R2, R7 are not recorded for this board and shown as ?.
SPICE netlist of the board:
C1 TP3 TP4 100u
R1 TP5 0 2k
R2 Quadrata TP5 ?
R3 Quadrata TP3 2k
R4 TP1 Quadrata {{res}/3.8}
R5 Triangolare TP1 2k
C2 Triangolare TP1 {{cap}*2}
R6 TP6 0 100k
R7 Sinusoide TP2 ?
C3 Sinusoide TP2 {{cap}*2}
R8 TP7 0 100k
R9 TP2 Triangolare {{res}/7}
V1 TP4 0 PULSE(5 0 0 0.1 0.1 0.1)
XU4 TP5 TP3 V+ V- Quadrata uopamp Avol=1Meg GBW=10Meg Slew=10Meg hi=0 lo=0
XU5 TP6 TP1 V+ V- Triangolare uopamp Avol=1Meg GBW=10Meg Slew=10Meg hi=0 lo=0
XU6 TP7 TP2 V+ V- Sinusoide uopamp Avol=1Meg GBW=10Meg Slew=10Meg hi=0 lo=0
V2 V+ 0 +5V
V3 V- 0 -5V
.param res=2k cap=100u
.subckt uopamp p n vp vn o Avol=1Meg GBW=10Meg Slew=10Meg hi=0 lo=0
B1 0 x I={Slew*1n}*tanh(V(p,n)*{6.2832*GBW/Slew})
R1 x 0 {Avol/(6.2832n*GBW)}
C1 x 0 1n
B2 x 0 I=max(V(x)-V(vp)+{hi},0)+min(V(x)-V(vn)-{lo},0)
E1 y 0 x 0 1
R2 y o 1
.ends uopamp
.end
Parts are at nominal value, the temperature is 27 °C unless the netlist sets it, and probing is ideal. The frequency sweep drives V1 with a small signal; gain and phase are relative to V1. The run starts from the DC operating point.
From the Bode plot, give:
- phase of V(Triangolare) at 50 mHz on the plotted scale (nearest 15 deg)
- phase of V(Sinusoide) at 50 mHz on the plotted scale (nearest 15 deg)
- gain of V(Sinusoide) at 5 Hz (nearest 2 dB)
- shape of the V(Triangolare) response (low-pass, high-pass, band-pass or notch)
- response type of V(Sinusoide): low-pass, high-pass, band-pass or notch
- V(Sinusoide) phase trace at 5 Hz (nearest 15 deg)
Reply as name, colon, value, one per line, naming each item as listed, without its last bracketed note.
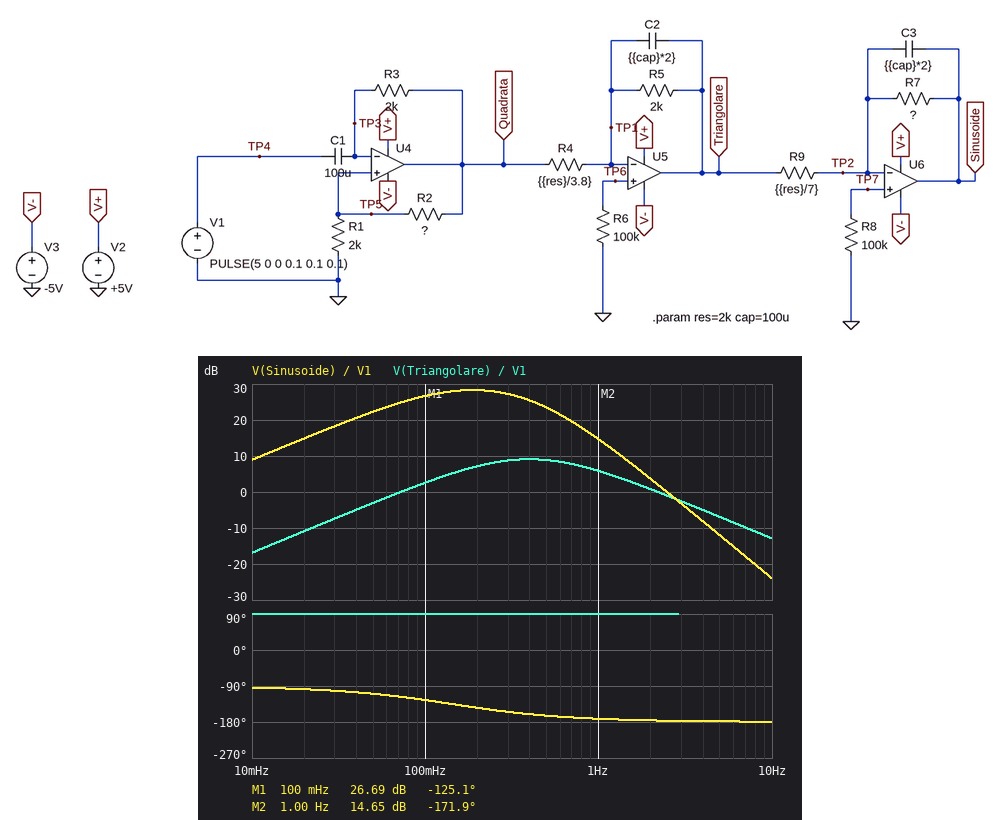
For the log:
phase of V(Triangolare) at 50 mHz on the plotted scale: 90 deg
phase of V(Sinusoide) at 50 mHz on the plotted scale: -105 deg
gain of V(Sinusoide) at 5 Hz: -12 dB
shape of the V(Triangolare) response: band-pass
response type of V(Sinusoide): low-pass, high-pass, band-pass or notch: band-pass
V(Sinusoide) phase trace at 5 Hz: -180 deg
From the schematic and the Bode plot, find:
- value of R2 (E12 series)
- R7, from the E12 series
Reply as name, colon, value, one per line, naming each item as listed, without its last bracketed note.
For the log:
value of R2: 1 kΩ
R7, from the E12 series: 5.6 kΩ
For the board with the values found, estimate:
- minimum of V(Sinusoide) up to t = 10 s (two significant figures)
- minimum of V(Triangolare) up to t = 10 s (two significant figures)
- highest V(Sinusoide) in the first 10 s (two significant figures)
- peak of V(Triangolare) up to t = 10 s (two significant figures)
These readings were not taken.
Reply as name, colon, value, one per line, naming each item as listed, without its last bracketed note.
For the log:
minimum of V(Sinusoide) up to t = 10 s: -5.0 V
minimum of V(Triangolare) up to t = 10 s: -5.0 V
highest V(Sinusoide) in the first 10 s: 5.0 V
peak of V(Triangolare) up to t = 10 s: 5.0 V
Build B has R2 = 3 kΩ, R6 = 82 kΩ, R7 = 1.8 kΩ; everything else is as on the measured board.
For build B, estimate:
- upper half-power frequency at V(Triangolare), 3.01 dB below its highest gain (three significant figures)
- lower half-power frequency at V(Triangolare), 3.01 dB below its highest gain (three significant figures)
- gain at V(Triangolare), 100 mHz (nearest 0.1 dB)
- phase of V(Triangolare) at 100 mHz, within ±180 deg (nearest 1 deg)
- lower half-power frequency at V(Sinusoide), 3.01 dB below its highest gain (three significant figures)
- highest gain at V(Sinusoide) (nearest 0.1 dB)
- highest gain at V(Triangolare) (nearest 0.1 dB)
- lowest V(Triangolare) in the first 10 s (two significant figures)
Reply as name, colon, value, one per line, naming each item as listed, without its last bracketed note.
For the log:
upper half-power frequency at V(Triangolare), 3.01 dB below its highest gain: 1.85 Hz
lower half-power frequency at V(Triangolare), 3.01 dB below its highest gain: 257 mHz
gain at V(Triangolare), 100 mHz: -2.3 dB
phase of V(Triangolare) at 100 mHz, within ±180 deg: 81 deg
lower half-power frequency at V(Sinusoide), 3.01 dB below its highest gain: 163 mHz
highest gain at V(Sinusoide): 20.0 dB
highest gain at V(Triangolare): 7.5 dB
lowest V(Triangolare) in the first 10 s: -5.0 V
